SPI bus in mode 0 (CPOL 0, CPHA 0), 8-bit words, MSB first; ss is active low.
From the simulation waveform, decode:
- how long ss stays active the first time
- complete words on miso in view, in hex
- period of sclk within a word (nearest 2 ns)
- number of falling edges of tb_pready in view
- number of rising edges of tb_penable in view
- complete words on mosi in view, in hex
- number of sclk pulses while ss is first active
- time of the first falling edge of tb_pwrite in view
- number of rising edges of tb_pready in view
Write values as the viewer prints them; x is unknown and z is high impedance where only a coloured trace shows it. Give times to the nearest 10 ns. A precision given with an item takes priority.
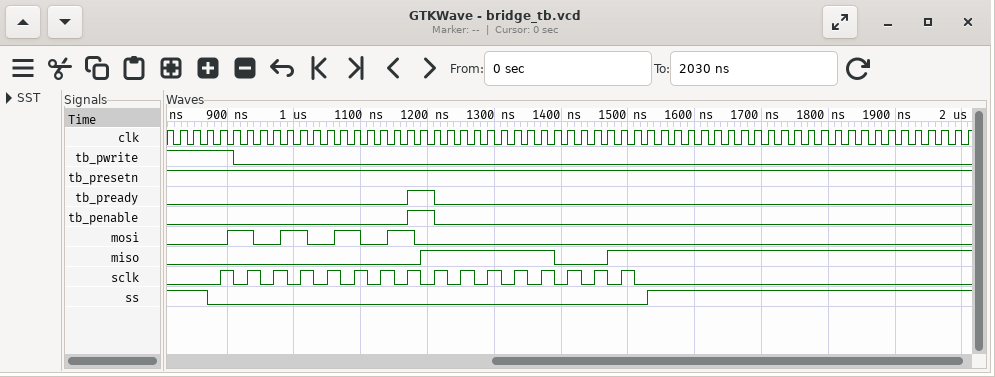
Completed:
660 ns
00, F9
40 ns
1
1
55, 00
16
910 ns
1
